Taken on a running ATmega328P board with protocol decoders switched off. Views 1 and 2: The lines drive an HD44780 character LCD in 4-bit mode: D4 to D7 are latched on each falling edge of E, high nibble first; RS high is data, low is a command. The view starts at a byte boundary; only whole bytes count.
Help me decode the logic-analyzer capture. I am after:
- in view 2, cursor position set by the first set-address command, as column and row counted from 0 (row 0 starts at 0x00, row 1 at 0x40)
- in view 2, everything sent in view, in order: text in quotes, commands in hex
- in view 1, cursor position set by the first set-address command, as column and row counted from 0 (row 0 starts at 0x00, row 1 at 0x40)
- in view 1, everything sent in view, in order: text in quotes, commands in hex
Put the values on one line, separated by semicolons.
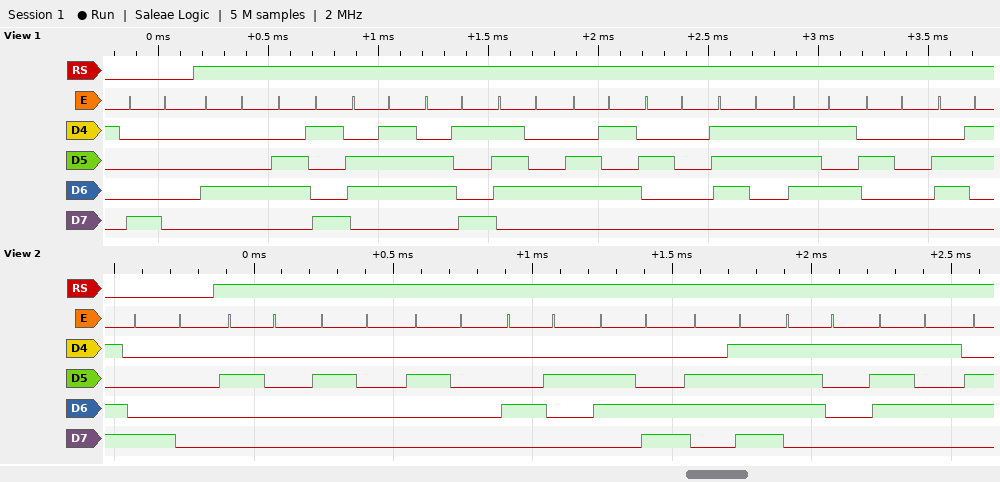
column 0, row 0; 0x80 "   Bloqu"; column 0, row 0; 0x80 "Digite su c"
